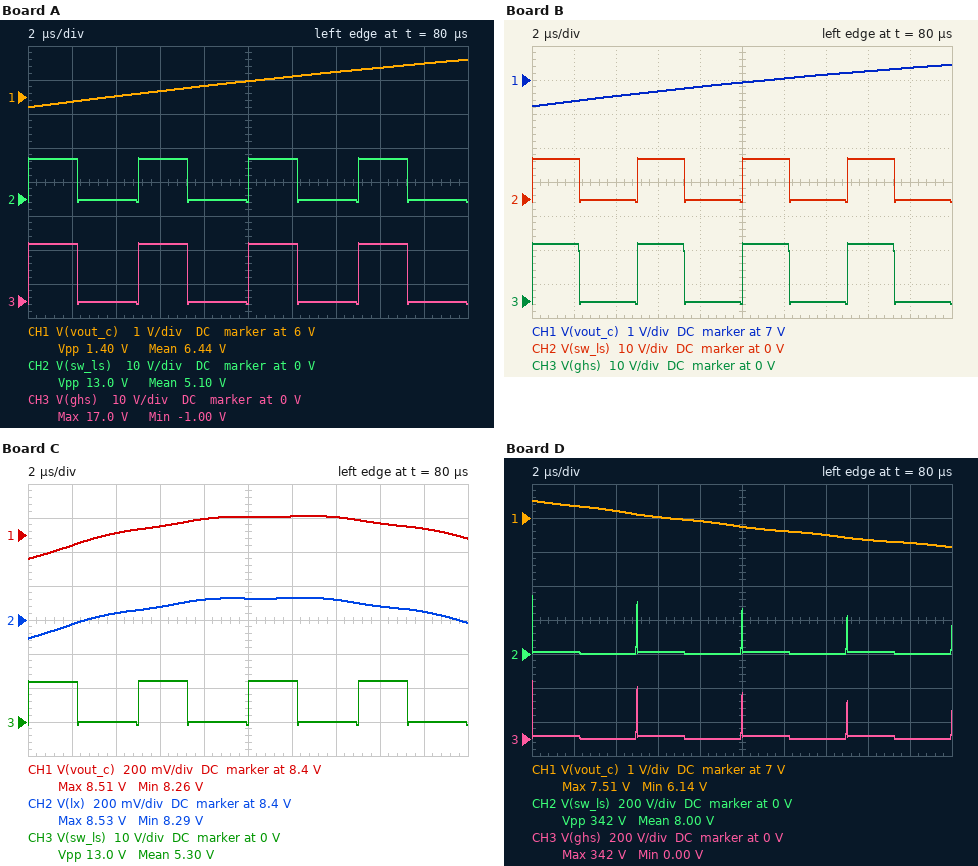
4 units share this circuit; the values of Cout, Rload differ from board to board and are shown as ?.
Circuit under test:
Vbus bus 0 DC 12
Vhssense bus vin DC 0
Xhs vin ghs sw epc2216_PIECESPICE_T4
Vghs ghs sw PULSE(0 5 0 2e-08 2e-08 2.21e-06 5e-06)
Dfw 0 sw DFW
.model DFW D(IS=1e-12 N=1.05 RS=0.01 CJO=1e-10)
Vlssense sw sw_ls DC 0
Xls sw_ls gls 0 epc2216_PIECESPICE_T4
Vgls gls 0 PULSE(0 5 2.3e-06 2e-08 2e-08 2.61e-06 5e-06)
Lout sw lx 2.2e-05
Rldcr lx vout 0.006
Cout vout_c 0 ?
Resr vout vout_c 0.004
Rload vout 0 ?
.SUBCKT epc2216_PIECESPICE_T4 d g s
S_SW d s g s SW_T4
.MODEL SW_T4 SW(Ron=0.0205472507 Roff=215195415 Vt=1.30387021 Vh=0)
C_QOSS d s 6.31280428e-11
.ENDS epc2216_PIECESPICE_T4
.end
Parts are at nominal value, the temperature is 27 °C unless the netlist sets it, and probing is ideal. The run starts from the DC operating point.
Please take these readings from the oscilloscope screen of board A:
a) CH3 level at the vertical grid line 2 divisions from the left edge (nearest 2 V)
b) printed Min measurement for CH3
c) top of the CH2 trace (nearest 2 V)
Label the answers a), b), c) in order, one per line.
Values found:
a) 0 V
b) -1.00 V
c) 12 V
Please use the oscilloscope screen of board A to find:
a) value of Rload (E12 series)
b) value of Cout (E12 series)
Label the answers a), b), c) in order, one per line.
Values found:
a) 1.5 Ω
b) 82 µF
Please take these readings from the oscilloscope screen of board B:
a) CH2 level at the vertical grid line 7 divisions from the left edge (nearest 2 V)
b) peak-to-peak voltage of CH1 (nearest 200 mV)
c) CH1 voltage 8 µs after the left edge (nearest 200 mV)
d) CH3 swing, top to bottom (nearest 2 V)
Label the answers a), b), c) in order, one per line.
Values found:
a) 0 V
b) 1.2 V
c) 6.8 V
d) 18 V
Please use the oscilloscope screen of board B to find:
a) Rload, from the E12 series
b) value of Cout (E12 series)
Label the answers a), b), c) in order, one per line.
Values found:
a) 1.5 Ω
b) 68 µF
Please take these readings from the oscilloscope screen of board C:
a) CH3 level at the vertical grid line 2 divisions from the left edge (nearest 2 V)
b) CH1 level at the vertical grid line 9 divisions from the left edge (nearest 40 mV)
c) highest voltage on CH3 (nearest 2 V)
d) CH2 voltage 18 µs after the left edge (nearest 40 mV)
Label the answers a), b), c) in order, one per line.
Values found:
a) 0 V
b) 8.44 V
c) 12 V
d) 8.44 V
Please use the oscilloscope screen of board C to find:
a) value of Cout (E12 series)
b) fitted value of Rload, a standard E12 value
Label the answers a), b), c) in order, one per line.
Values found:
a) 39 µF
b) 2.7 Ω
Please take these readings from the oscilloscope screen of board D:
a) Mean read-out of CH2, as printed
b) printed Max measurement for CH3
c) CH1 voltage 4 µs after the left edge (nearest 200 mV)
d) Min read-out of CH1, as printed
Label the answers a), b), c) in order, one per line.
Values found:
a) 8.00 V
b) 342 V
c) 7.2 V
d) 6.14 V
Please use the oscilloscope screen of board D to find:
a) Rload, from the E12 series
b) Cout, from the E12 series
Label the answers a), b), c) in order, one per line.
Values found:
a) 8.2 Ω
b) 15 µF
